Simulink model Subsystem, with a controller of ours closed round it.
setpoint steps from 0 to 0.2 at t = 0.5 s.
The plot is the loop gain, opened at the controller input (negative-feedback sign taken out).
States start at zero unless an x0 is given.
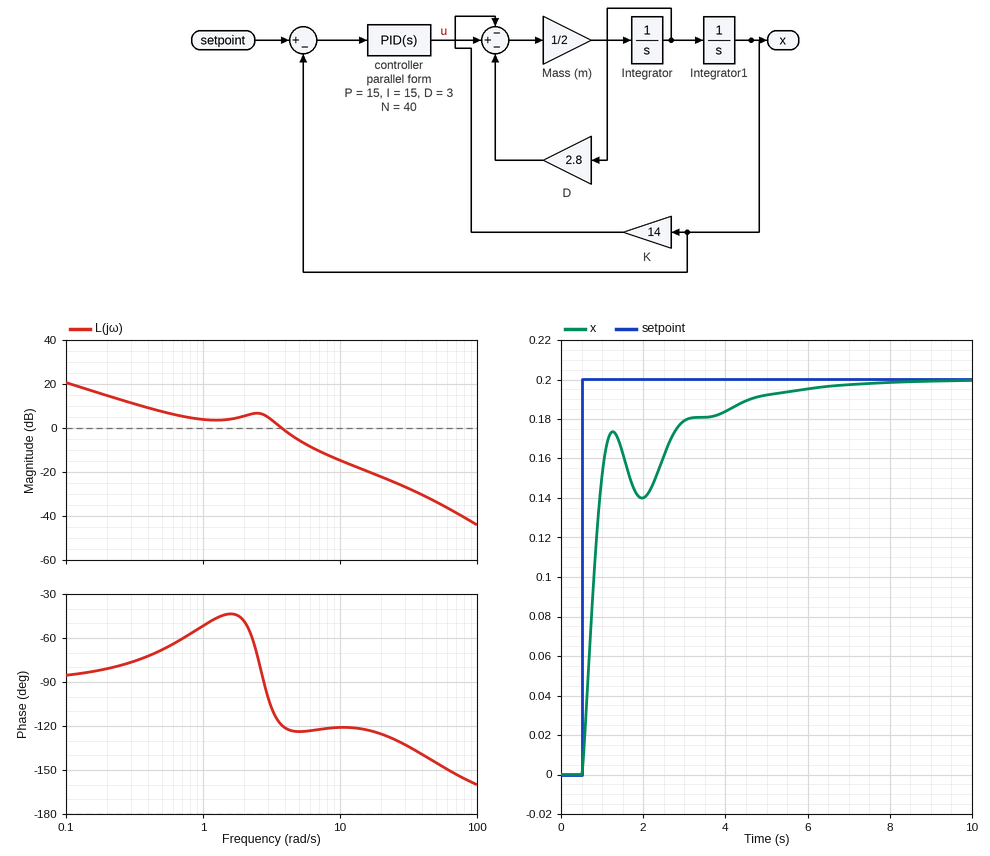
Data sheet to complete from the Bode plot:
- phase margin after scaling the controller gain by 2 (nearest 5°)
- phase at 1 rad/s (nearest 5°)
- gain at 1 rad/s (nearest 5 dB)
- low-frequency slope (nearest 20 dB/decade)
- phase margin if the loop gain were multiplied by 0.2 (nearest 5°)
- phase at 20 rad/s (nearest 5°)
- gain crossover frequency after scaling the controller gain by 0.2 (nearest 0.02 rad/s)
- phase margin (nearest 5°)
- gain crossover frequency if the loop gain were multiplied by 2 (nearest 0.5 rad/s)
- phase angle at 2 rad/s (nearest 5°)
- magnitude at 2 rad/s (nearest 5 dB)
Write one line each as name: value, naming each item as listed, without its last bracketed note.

phase margin after scaling the controller gain by 2: 55°
phase at 1 rad/s: -50°
gain at 1 rad/s: 5 dB
low-frequency slope: -20 dB/decade
phase margin if the loop gain were multiplied by 0.2: 100°
phase at 20 rad/s: -125°
gain crossover frequency after scaling the controller gain by 0.2: 0.22 rad/s
phase margin: 60°
gain crossover frequency if the loop gain were multiplied by 2: 5.0 rad/s
phase angle at 2 rad/s: -50°
magnitude at 2 rad/s: 5 dB
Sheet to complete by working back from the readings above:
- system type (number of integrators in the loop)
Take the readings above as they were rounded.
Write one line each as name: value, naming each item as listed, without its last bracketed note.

system type: 1
